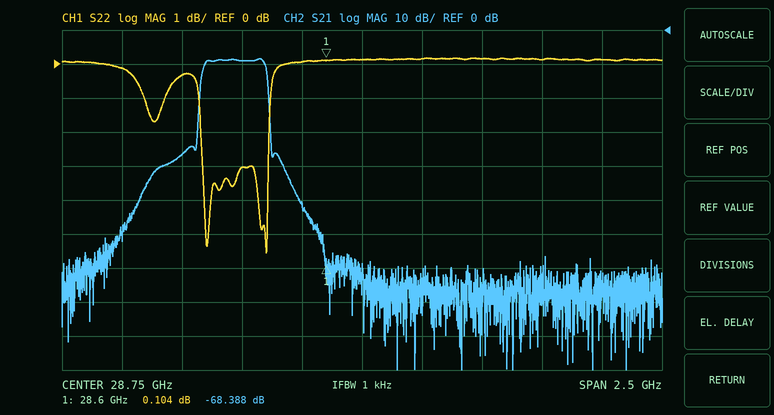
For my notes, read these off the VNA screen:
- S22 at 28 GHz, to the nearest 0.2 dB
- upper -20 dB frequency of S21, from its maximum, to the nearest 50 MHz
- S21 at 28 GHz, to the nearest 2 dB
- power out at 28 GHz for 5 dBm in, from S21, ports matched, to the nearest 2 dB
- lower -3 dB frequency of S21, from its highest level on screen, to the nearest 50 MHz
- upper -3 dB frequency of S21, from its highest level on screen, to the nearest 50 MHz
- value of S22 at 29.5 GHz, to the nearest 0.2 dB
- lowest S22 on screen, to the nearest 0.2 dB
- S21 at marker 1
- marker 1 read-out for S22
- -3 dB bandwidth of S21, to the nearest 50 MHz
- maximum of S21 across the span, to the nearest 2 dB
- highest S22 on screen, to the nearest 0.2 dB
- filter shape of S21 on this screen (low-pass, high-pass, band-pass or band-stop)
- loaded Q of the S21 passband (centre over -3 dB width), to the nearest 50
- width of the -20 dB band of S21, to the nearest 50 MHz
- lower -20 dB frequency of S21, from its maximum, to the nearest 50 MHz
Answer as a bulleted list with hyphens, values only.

- -0.4 dB
- 28.35 GHz
- -36 dB
- -32 dBm
- 28.10 GHz
- 28.35 GHz
- 0.2 dB
- -5.6 dB
- -68.388 dB
- 0.104 dB
- 250 MHz
- -8 dB
- 0.2 dB
- band-pass
- 100
- 300 MHz
- 28.05 GHz
